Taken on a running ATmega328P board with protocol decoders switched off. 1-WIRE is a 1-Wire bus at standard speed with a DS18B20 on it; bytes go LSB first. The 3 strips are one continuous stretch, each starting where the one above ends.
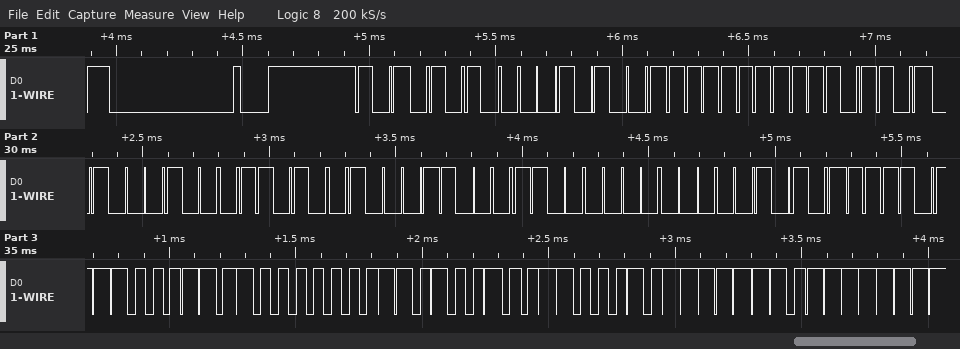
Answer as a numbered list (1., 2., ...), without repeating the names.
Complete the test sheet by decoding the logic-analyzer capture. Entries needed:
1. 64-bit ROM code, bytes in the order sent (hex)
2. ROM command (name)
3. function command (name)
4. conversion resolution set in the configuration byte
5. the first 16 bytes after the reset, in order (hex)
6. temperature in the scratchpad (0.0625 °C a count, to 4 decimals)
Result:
1. 28 FF B7 22 96 18 03 A0
2. Match ROM
3. Read Scratchpad
4. 12 bits
5. 55 28 FF B7 22 96 18 03 A0 BE 63 01 4B 46 7F FF
6. 22.1875 °C
